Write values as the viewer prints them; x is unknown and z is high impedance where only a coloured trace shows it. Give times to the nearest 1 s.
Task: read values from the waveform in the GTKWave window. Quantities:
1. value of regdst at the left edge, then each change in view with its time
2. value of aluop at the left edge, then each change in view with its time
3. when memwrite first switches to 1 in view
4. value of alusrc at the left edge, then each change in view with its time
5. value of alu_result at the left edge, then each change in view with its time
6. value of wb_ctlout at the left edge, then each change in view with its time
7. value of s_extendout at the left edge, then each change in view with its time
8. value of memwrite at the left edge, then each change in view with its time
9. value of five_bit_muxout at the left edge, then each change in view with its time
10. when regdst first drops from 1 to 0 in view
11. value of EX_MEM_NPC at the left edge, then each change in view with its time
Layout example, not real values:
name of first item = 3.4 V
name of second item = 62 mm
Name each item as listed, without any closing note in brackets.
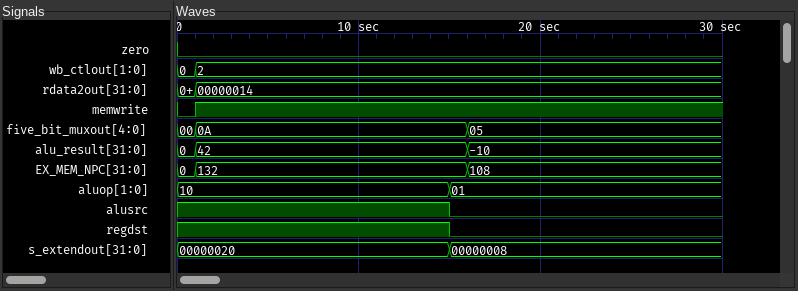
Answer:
value of regdst at the left edge, then each change in view with its time = 1, 0 at 15 s
value of aluop at the left edge, then each change in view with its time = 10, 01 at 15 s
when memwrite first switches to 1 in view = 1 s
value of alusrc at the left edge, then each change in view with its time = 1, 0 at 15 s
value of alu_result at the left edge, then each change in view with its time = 0, 42 at 1 s, -10 at 16 s
value of wb_ctlout at the left edge, then each change in view with its time = 0, 2 at 1 s
value of s_extendout at the left edge, then each change in view with its time = 00000020, 00000008 at 15 s
value of memwrite at the left edge, then each change in view with its time = 0, 1 at 1 s
value of five_bit_muxout at the left edge, then each change in view with its time = 00, 0A at 1 s, 05 at 16 s
when regdst first drops from 1 to 0 in view = 15 s
value of EX_MEM_NPC at the left edge, then each change in view with its time = 0, 132 at 1 s, 108 at 16 s
